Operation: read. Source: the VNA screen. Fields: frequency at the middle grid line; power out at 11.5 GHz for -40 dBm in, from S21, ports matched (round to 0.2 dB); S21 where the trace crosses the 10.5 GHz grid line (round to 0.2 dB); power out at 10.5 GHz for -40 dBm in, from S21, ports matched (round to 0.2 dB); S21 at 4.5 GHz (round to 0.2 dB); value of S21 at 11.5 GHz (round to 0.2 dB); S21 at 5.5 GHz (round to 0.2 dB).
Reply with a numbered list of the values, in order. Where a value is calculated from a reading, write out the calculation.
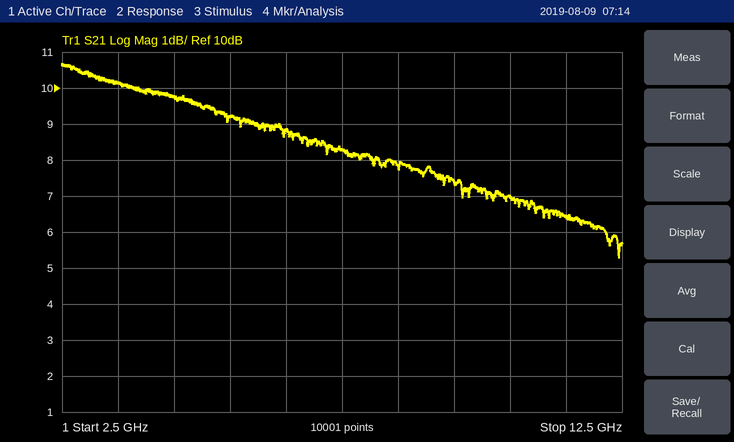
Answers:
1. 7.5 GHz
2. -40 dBm + (6.4 dB) = -33.6 dBm
3. 7.0 dB
4. -40 dBm + (7.0 dB) = -33.0 dBm
5. 9.8 dB
6. 6.4 dB
7. 9.2 dB
